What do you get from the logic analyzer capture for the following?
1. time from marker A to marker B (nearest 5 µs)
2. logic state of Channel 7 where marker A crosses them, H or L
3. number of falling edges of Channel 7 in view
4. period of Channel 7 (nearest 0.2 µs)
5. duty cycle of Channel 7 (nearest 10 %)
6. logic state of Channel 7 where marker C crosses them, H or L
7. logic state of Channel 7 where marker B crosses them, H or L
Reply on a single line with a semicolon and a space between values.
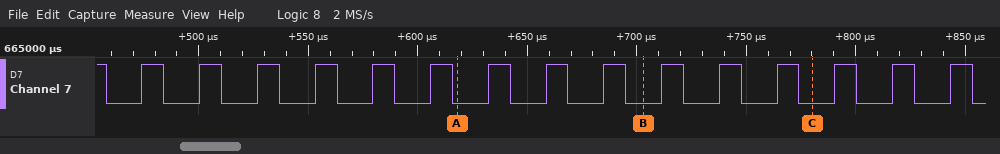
85 µs; Channel 7=L; 16; 26.4 µs; 40 %; Channel 7=L; Channel 7=L
